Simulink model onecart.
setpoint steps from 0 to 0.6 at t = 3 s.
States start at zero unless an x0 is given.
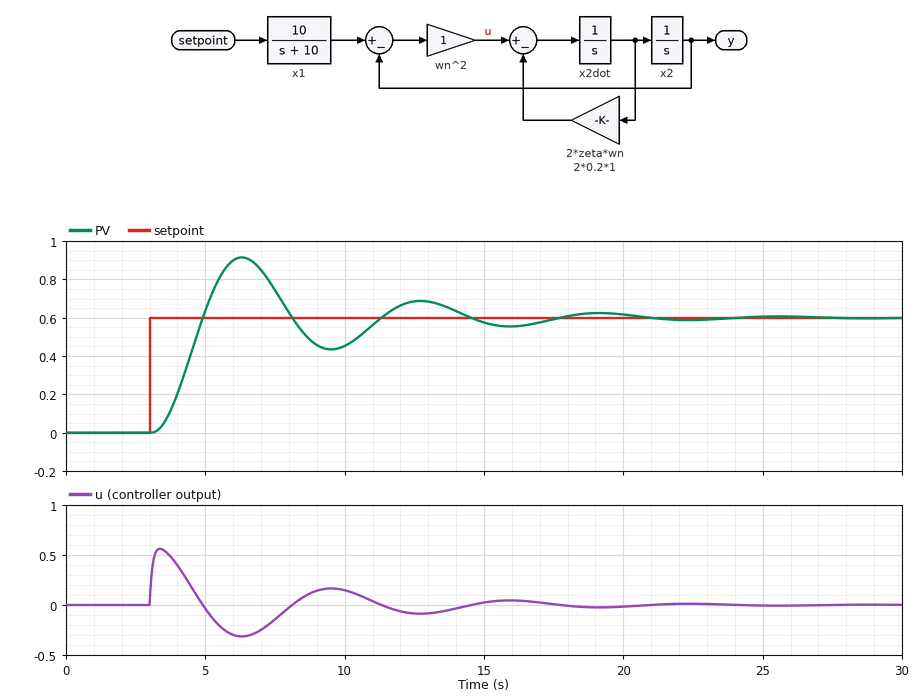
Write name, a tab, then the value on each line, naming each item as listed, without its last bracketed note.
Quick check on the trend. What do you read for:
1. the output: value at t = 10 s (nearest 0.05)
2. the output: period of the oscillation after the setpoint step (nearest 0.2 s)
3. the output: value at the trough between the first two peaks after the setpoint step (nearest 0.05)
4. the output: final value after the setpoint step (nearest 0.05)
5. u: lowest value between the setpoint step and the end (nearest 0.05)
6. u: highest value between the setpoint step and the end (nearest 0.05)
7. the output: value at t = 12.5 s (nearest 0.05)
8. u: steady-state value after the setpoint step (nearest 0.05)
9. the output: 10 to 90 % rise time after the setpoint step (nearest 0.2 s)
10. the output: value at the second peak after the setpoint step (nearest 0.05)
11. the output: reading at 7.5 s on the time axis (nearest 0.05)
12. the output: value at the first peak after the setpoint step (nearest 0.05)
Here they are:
the output: value at t = 10 s	0.45
the output: period of the oscillation after the setpoint step	6.4 s
the output: value at the trough between the first two peaks after the setpoint step	0.45
the output: final value after the setpoint step	0.60
u: lowest value between the setpoint step and the end	-0.30
u: highest value between the setpoint step and the end	0.55
the output: value at t = 12.5 s	0.70
u: steady-state value after the setpoint step	0.00
the output: 10 to 90 % rise time after the setpoint step	1.2 s
the output: value at the second peak after the setpoint step	0.70
the output: reading at 7.5 s on the time axis	0.75
the output: value at the first peak after the setpoint step	0.90
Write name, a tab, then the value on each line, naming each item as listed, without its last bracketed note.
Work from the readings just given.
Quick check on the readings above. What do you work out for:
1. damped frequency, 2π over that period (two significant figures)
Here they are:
damped frequency, 2π over that period	0.98 rad/s
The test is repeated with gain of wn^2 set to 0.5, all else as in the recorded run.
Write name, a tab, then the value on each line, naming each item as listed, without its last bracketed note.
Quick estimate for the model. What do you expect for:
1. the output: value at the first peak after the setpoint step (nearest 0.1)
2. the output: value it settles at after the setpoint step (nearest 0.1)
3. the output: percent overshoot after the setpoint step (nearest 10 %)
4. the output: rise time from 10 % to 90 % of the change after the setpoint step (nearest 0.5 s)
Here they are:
the output: value at the first peak after the setpoint step	0.8
the output: value it settles at after the setpoint step	0.6
the output: percent overshoot after the setpoint step	40 %
the output: rise time from 10 % to 90 % of the change after the setpoint step	2.0 s
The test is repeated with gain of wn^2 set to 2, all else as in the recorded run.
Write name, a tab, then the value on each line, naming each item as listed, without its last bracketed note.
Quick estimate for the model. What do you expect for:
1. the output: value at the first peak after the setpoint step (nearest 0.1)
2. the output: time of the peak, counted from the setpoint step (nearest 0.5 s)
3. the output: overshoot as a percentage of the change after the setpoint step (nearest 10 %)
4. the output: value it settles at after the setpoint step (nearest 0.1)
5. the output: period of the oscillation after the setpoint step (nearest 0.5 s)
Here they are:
the output: value at the first peak after the setpoint step	1.0
the output: time of the peak, counted from the setpoint step	2.5 s
the output: overshoot as a percentage of the change after the setpoint step	60 %
the output: value it settles at after the setpoint step	0.6
the output: period of the oscillation after the setpoint step	4.5 s
